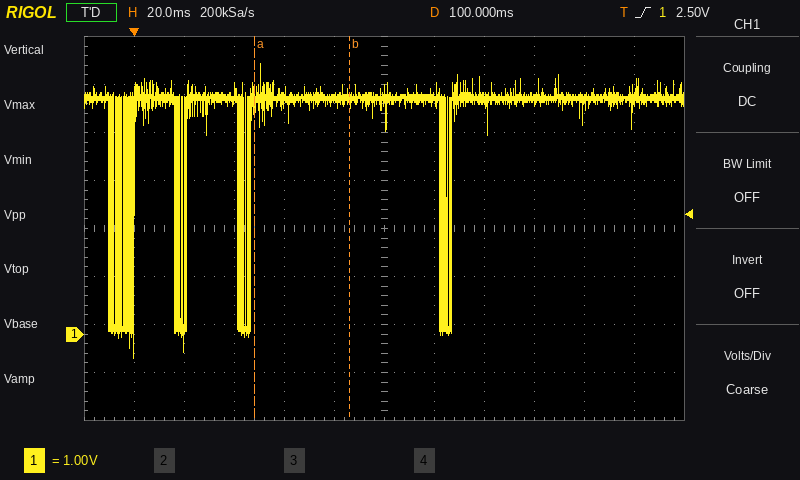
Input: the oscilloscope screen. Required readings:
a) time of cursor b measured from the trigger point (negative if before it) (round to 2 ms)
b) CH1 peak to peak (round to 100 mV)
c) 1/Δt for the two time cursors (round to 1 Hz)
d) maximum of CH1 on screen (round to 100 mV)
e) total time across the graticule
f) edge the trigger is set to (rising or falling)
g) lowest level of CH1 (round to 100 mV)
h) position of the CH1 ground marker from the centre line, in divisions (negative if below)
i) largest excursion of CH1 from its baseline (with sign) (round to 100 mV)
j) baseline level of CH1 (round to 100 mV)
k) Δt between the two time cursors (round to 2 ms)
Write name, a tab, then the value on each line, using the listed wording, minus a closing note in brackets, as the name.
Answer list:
time of cursor b measured from the trigger point (negative if before it)	+86 ms
CH1 peak to peak	6.1 V
1/Δt for the two time cursors	26 Hz
maximum of CH1 on screen	5.6 V
total time across the graticule	240 ms
edge the trigger is set to	rising
lowest level of CH1	-500 mV
position of the CH1 ground marker from the centre line, in divisions	-2.2 div
largest excursion of CH1 from its baseline (with sign)	-5.4 V
baseline level of CH1	4.9 V
Δt between the two time cursors	38 ms
